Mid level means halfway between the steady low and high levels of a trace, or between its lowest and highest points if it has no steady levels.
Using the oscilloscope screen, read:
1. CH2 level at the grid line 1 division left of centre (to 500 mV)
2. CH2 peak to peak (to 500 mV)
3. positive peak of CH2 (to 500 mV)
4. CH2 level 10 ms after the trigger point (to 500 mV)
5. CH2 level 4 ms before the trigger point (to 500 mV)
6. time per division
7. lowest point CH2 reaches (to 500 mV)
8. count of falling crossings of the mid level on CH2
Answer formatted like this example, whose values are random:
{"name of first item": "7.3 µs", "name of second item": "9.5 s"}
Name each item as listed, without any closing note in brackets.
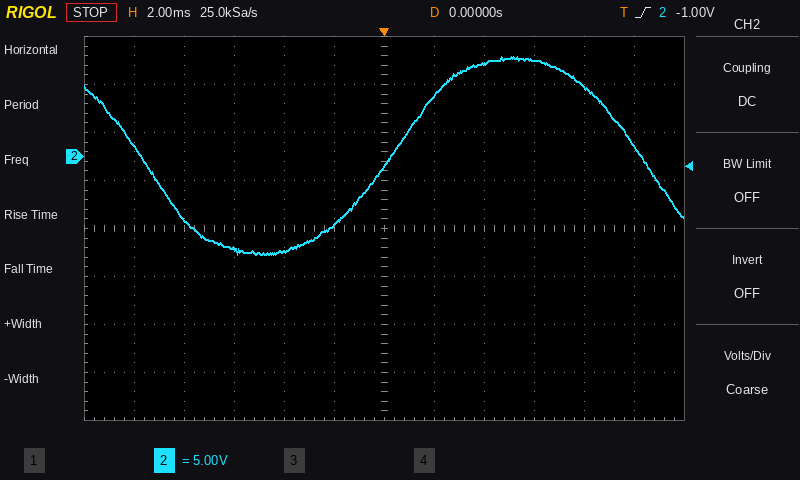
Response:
{"CH2 level at the grid line 1 division left of centre": "-7.0 V", "CH2 peak to peak": "20.5 V", "positive peak of CH2": "10.5 V", "CH2 level 10 ms after the trigger point": "1.0 V", "CH2 level 4 ms before the trigger point": "-10.0 V", "time per division": "2 ms", "lowest point CH2 reaches": "-10.0 V", "count of falling crossings of the mid level on CH2": "2"}
